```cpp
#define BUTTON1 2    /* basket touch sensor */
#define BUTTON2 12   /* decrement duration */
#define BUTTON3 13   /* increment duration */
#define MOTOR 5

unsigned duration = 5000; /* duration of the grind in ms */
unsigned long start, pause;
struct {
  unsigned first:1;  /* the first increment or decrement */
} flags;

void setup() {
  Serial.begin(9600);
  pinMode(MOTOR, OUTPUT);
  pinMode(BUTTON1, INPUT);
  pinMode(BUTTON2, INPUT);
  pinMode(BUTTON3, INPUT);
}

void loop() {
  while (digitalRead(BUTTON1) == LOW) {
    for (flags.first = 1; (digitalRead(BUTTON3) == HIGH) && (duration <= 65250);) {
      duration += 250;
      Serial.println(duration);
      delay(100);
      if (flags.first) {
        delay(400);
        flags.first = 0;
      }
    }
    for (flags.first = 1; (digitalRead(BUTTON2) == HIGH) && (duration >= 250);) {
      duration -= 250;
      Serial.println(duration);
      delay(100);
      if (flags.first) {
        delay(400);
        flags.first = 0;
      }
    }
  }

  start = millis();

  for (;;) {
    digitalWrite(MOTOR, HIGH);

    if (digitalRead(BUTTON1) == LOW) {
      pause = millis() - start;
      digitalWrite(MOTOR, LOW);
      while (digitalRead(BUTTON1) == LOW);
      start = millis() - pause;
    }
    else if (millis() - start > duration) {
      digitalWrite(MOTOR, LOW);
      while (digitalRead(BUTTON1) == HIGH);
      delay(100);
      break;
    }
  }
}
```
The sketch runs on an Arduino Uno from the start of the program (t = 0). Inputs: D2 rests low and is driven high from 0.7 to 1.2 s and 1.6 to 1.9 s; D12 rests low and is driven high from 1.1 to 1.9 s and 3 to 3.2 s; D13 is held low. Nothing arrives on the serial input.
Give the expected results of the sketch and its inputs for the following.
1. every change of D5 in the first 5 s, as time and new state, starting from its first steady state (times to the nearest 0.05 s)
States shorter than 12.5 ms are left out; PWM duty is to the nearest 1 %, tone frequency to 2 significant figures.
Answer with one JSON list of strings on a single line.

["0 s low; 0.7 s high; 1.2 s low; 1.6 s high; 1.9 s low"]
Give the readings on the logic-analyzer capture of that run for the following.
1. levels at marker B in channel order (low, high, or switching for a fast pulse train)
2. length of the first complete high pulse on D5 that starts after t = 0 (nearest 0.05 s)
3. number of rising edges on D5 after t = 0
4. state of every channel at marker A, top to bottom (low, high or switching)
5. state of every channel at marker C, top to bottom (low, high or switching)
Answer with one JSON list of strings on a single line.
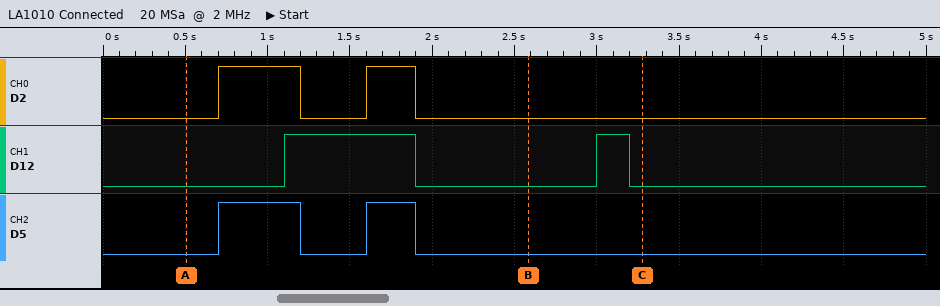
["D2 low, D12 low, D5 low", "0.50 s", "2", "D2 low, D12 low, D5 low", "D2 low, D12 low, D5 low"]
